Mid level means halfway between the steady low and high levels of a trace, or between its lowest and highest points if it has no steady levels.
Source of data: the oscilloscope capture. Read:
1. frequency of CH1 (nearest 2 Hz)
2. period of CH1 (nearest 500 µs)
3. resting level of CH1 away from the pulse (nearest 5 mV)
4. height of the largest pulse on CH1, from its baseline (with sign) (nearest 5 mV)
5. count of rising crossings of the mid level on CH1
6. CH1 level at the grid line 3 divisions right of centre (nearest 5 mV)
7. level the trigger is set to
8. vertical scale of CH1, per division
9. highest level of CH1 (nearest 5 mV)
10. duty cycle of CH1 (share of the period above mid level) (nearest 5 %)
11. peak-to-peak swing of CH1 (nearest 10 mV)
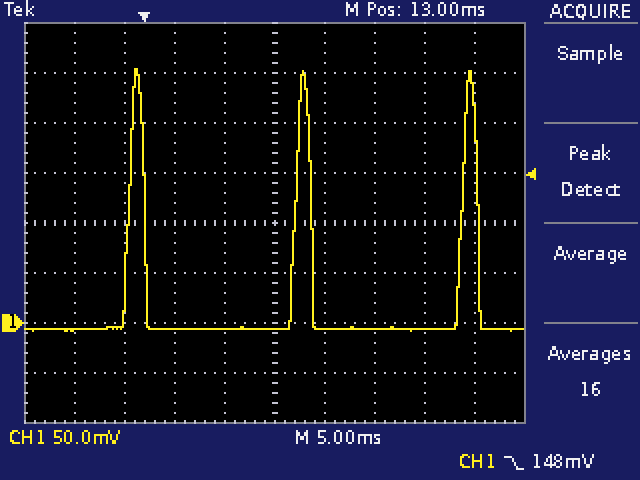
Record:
60 Hz
16.5 ms
-5 mV
+260 mV
3
-5 mV
148 mV
50 mV
255 mV
10 %
260 mV
